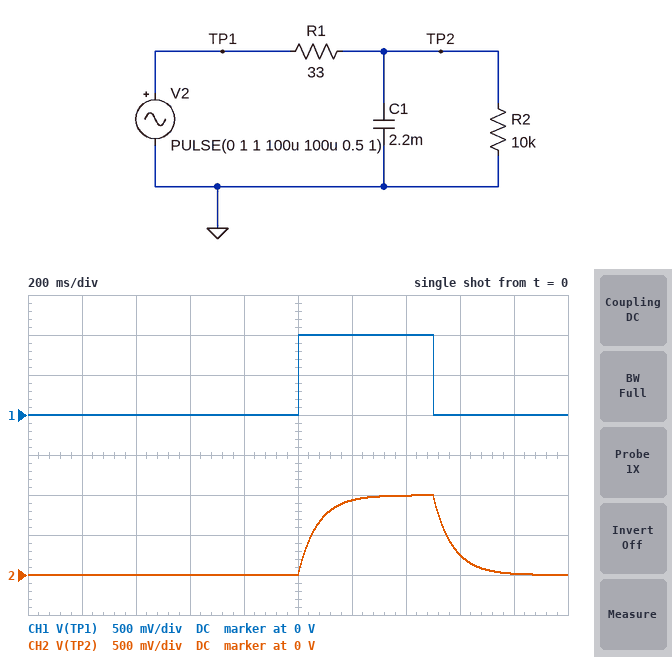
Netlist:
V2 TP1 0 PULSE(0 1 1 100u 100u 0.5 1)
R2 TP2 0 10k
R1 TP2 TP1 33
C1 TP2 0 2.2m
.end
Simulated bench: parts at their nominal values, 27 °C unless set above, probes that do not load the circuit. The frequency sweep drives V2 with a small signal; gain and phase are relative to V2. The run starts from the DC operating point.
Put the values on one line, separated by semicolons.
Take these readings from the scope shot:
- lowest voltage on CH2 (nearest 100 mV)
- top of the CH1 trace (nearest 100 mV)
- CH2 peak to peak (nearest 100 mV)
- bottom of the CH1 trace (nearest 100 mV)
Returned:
0 V; 1.0 V; 1.0 V; 0 V
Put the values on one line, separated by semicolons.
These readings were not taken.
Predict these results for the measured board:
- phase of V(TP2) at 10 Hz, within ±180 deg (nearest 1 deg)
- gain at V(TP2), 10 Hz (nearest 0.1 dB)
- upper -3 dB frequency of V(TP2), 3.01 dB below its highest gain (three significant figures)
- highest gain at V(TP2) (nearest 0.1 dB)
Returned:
-78 deg; -13.4 dB; 2.20 Hz; 0 dB
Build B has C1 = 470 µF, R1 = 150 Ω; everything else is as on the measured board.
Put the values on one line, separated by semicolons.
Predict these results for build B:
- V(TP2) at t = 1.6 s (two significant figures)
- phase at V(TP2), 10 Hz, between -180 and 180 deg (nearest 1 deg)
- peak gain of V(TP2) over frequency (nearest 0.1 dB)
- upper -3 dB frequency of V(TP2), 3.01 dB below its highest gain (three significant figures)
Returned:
230 mV; -77 deg; -0.1 dB; 2.29 Hz
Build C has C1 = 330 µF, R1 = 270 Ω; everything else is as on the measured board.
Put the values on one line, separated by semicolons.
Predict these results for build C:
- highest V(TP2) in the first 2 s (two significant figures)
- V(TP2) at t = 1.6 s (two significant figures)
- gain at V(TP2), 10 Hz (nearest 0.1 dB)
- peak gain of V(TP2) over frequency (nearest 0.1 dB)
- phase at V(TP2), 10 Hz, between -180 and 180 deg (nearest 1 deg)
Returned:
970 mV; 310 mV; -15.1 dB; -0.2 dB; -80 deg
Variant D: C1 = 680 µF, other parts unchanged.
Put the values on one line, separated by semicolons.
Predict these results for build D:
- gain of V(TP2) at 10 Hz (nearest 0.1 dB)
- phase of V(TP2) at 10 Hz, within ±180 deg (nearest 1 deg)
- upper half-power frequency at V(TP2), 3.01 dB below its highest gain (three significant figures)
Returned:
-4.8 dB; -55 deg; 7.12 Hz
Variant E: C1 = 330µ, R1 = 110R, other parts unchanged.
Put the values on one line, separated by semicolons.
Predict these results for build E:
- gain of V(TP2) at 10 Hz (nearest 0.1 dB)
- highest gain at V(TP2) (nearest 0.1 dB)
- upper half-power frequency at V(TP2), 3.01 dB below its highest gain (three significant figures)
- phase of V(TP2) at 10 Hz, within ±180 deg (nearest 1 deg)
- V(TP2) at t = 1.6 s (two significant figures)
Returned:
-7.9 dB; -0.1 dB; 4.43 Hz; -66 deg; 61 mV
